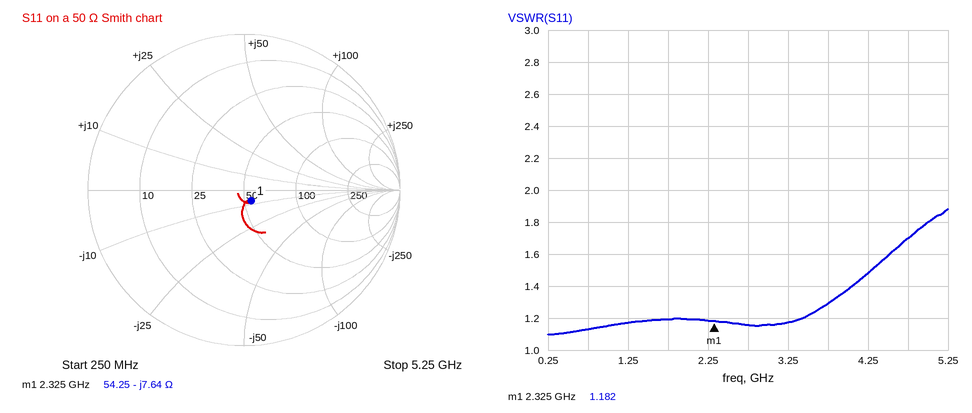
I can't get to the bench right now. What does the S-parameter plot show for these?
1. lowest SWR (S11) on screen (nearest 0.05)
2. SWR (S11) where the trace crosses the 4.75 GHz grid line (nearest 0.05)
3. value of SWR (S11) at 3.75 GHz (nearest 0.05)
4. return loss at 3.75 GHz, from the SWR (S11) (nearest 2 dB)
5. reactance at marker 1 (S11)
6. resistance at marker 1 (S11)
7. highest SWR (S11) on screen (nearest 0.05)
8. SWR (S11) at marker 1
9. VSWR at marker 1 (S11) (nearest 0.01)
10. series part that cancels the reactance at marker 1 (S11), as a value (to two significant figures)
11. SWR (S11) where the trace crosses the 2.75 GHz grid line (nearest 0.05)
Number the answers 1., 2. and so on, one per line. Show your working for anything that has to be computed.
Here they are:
1. 1.10
2. 1.70
3. 1.30
4. −20 log10((1.3 − 1)/(1.3 + 1)) ≈ 18 dB
5. -7.64 Ω
6. 54.25 Ω
7. 1.90
8. 1.182
9. 1.18
10. L = 7.64 Ω/(2π × 2.325 GHz) ≈ 523 pH, so 520 pH to two significant figures
11. 1.15
